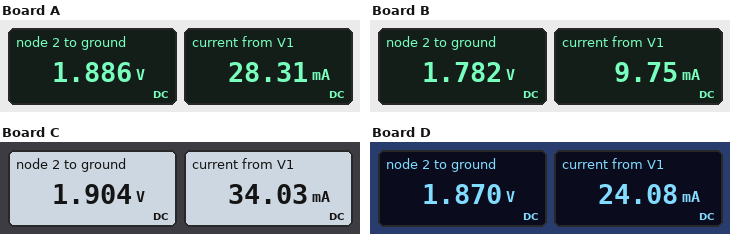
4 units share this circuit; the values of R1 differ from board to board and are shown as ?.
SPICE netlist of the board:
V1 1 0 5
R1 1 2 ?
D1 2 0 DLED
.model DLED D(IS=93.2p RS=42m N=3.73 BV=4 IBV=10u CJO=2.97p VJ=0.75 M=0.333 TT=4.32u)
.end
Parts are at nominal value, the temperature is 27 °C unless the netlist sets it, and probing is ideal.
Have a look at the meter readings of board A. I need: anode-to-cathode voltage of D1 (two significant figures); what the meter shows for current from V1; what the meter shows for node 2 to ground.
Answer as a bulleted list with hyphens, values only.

- 1.9 V
- 28.31 mA
- 1.886 V
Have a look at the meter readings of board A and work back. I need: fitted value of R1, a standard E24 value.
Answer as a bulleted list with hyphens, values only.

- 110 Ω
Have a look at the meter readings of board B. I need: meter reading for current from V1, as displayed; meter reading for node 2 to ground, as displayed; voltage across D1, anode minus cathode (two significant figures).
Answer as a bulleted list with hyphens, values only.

- 9.75 mA
- 1.782 V
- 1.8 V
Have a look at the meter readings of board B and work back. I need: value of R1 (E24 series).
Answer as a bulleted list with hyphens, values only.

- 330 Ω
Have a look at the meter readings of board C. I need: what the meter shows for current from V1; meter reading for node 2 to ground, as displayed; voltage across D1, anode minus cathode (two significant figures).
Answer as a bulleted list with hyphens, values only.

- 34.03 mA
- 1.904 V
- 1.9 V
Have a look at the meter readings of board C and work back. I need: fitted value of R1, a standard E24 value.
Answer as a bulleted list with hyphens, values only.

- 91 Ω
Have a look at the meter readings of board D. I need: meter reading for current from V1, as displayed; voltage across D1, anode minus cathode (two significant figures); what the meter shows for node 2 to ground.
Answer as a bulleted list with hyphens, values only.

- 24.08 mA
- 1.9 V
- 1.870 V
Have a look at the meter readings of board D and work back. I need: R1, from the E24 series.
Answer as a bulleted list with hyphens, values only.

- 130 Ω
